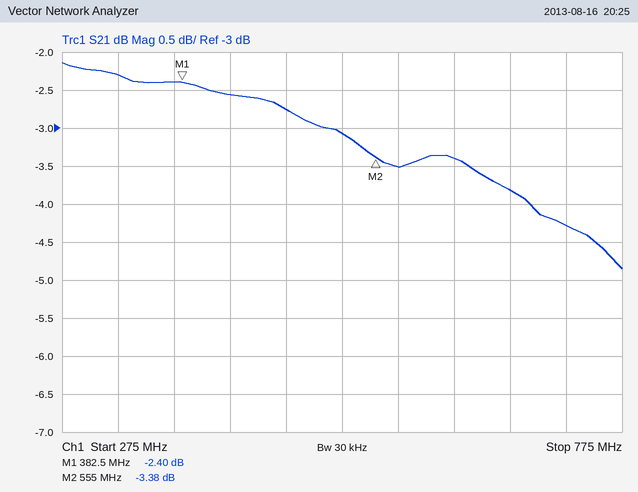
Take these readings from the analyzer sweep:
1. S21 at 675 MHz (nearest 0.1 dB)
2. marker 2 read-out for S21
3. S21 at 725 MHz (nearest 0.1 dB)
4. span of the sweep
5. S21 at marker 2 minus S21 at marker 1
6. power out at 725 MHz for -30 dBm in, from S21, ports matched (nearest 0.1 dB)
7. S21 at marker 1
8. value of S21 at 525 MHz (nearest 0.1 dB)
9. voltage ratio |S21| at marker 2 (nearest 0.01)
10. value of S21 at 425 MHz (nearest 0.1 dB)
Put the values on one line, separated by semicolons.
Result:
-3.8 dB; -3.38 dB; -4.3 dB; 500 MHz; -0.98 dB; -34.3 dBm; -2.40 dB; -3.1 dB; 0.68; -2.6 dB
